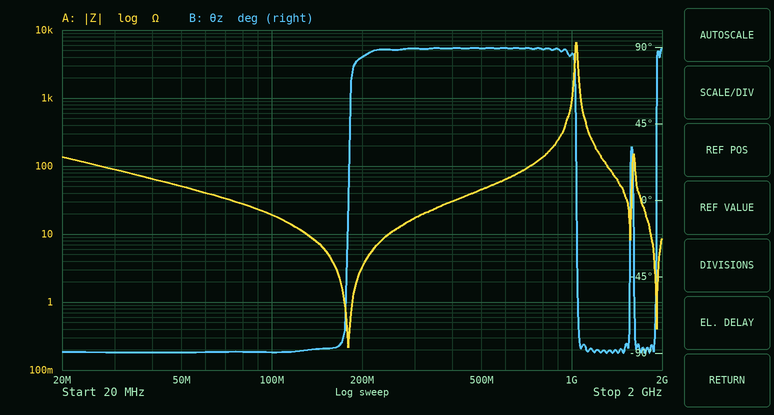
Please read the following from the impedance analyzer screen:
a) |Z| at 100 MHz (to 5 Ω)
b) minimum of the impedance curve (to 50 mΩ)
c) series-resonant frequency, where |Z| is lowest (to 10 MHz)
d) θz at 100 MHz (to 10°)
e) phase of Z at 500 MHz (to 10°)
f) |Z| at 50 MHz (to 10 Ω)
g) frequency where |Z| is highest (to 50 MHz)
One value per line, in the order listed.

20 Ω
200 mΩ
180 MHz
-90°
90°
50 Ω
1.05 GHz
